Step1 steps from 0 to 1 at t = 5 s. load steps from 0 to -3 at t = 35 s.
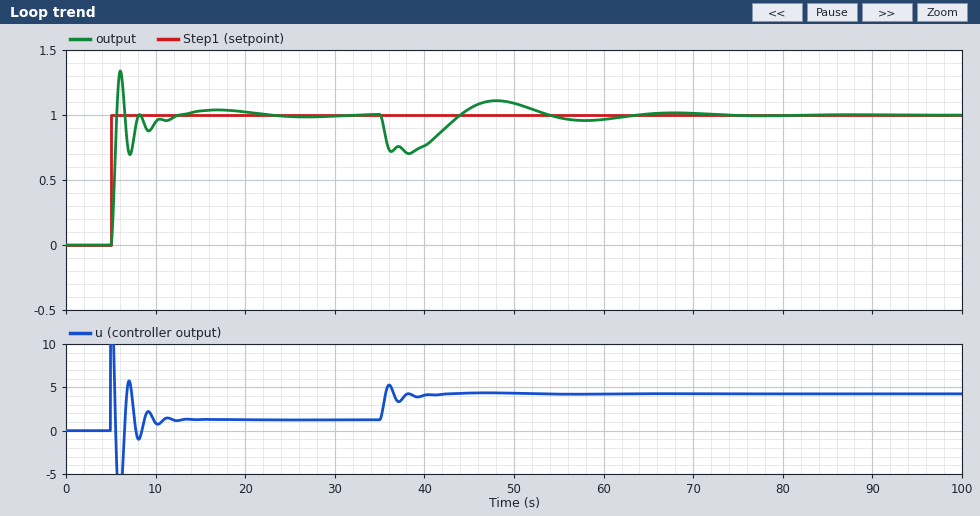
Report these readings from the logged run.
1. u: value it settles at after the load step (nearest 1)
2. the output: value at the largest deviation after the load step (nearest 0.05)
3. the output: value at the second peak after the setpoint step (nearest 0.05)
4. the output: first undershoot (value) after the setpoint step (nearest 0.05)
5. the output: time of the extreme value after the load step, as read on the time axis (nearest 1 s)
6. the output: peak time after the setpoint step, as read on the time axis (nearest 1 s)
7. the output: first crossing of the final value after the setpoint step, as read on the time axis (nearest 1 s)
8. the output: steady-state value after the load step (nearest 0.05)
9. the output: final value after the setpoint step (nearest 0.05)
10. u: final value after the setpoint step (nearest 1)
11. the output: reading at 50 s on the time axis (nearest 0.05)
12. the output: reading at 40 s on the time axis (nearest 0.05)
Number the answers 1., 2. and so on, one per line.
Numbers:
1. 4
2. 0.70
3. 1.00
4. 0.70
5. 38 s
6. 6 s
7. 6 s
8. 1.00
9. 1.00
10. 1
11. 1.10
12. 0.75
